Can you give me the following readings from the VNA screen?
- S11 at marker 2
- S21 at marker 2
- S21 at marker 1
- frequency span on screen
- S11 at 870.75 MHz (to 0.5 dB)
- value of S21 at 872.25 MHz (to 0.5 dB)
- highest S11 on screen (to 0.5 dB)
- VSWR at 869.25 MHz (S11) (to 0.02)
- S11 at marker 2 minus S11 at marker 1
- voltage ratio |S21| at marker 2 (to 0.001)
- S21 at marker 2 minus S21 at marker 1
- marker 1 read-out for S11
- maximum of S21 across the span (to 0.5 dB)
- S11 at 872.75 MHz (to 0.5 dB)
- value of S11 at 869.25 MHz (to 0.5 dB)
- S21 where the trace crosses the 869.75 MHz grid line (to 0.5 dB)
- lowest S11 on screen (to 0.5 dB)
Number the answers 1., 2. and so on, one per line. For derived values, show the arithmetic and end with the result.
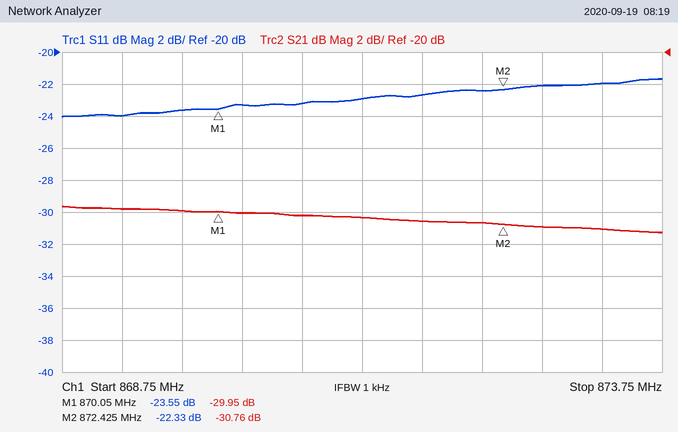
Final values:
1. -22.33 dB
2. -30.76 dB
3. -29.95 dB
4. 5 MHz
5. -23.0 dB
6. -30.5 dB
7. -21.5 dB
8. |Γ| = 10^(-24/20) = 0.0631; VSWR = (1 + 0.0631)/(1 − 0.0631) ≈ 1.13, so 1.14 to the nearest 0.02
9. -22.33 − (-23.55) = 1.22 dB
10. 10^(-30.76/20) ≈ 0.029
11. -30.76 − (-29.95) = -0.81 dB
12. -23.55 dB
13. -29.5 dB
14. -22.0 dB
15. -24.0 dB
16. -30.0 dB
17. -24.0 dB
